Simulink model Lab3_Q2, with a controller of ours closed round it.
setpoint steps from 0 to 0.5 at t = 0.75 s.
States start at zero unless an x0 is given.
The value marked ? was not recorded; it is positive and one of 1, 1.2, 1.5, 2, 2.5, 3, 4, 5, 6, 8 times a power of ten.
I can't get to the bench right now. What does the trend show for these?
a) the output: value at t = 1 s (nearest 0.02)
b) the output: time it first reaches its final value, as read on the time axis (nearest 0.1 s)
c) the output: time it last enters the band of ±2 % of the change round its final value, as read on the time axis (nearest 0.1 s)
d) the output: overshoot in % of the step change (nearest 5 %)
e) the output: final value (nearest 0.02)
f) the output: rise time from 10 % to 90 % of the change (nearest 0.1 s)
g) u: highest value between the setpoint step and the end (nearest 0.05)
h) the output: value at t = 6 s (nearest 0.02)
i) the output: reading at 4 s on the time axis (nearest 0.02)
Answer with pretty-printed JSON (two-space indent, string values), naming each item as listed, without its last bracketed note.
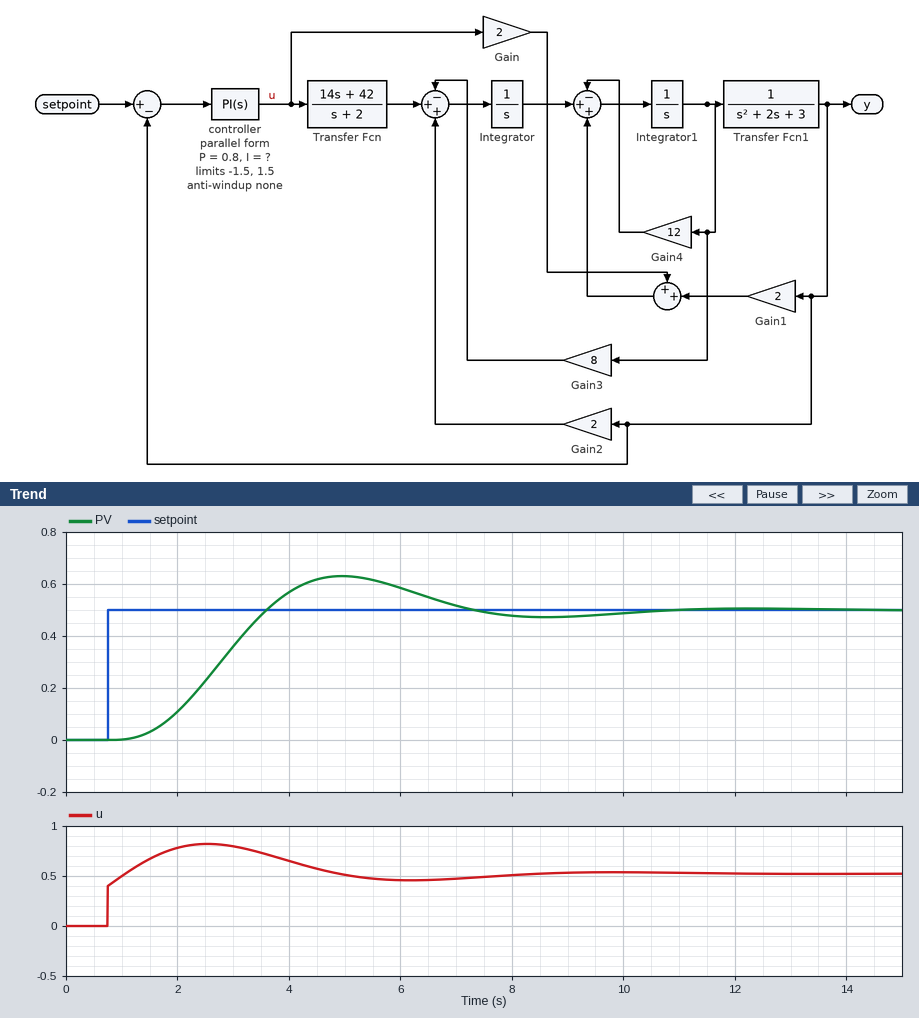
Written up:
{
  "the output: value at t = 1 s": "0.00",
  "the output: time it first reaches its final value, as read on the time axis": "3.6 s",
  "the output: time it last enters the band of ±2 % of the change round its final value, as read on the time axis": "10.2 s",
  "the output: overshoot in % of the step change": "25 %",
  "the output: final value": "0.50",
  "the output: rise time from 10 % to 90 % of the change": "1.7 s",
  "u: highest value between the setpoint step and the end": "0.80",
  "the output: value at t = 6 s": "0.58",
  "the output: reading at 4 s on the time axis": "0.56"
}
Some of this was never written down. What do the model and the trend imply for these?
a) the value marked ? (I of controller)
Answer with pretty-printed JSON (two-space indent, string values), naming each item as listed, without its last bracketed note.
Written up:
{
  "the value marked ?": "0.8"
}
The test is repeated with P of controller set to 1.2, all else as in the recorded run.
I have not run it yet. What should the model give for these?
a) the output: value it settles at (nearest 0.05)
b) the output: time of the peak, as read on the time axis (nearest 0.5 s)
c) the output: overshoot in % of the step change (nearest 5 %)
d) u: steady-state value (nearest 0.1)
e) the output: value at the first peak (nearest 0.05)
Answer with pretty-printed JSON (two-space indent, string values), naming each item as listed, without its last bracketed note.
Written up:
{
  "the output: value it settles at": "0.50",
  "the output: time of the peak, as read on the time axis": "4.5 s",
  "the output: overshoot in % of the step change": "20 %",
  "u: steady-state value": "0.5",
  "the output: value at the first peak": "0.60"
}
